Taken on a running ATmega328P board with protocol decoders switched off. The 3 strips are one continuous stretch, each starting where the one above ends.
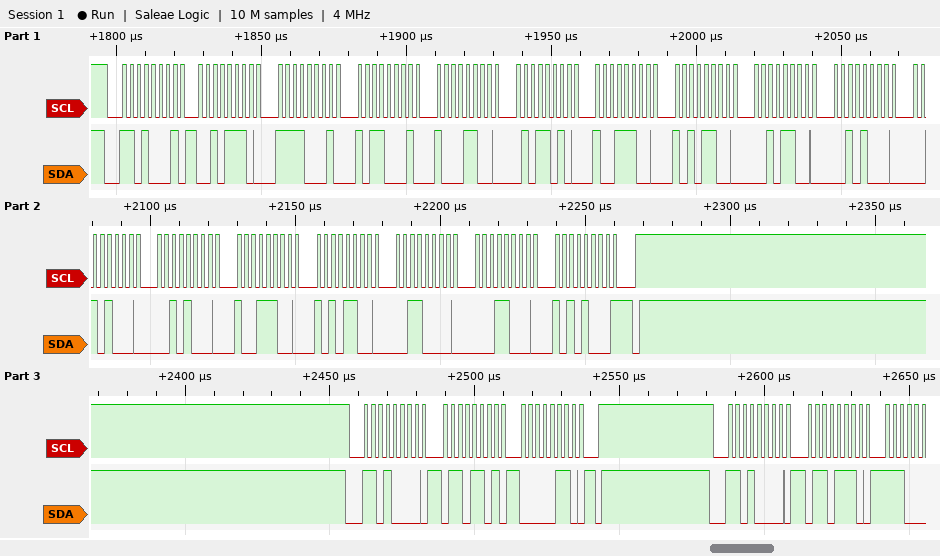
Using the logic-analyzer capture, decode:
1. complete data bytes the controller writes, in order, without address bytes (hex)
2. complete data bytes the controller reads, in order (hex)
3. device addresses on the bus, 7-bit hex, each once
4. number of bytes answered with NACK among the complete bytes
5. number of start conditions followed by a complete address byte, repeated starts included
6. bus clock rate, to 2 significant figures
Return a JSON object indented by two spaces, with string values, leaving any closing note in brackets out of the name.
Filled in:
{
  "complete data bytes the controller writes, in order, without address bytes": "6D 06 6E",
  "complete data bytes the controller reads, in order": "2E F1 B1 8C 5A 9C AC 2C 28 28 28 9C AC 30 18 A8",
  "device addresses on the bus, 7-bit hex, each once": "0x68",
  "number of bytes answered with NACK among the complete bytes": "1",
  "number of start conditions followed by a complete address byte, repeated starts included": "3",
  "bus clock rate, to 2 significant figures": "400 kHz"
}
